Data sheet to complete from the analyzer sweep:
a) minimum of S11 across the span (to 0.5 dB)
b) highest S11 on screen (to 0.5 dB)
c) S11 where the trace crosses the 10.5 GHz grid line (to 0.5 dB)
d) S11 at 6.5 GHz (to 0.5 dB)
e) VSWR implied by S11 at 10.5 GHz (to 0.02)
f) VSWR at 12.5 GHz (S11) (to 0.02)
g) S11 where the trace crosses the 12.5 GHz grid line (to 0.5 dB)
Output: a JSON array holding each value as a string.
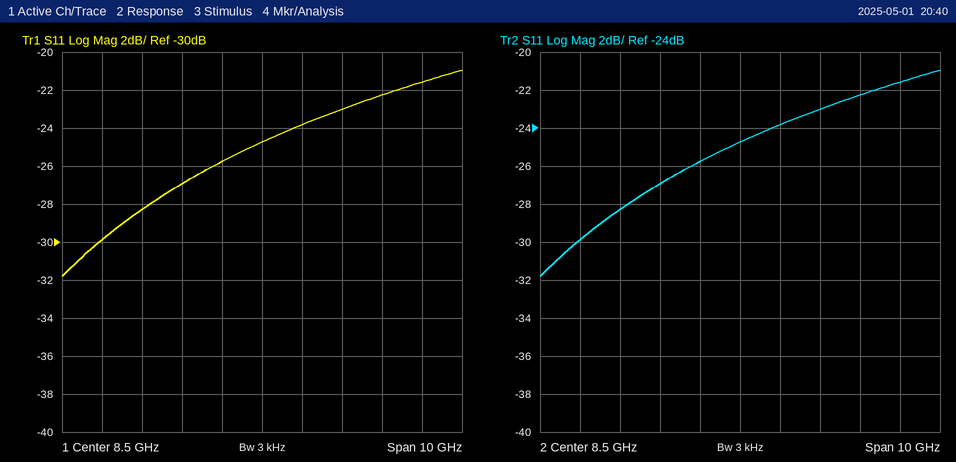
["-32.0 dB", "-21.0 dB", "-23.0 dB", "-27.0 dB", "1.16", "1.18", "-21.5 dB"]
